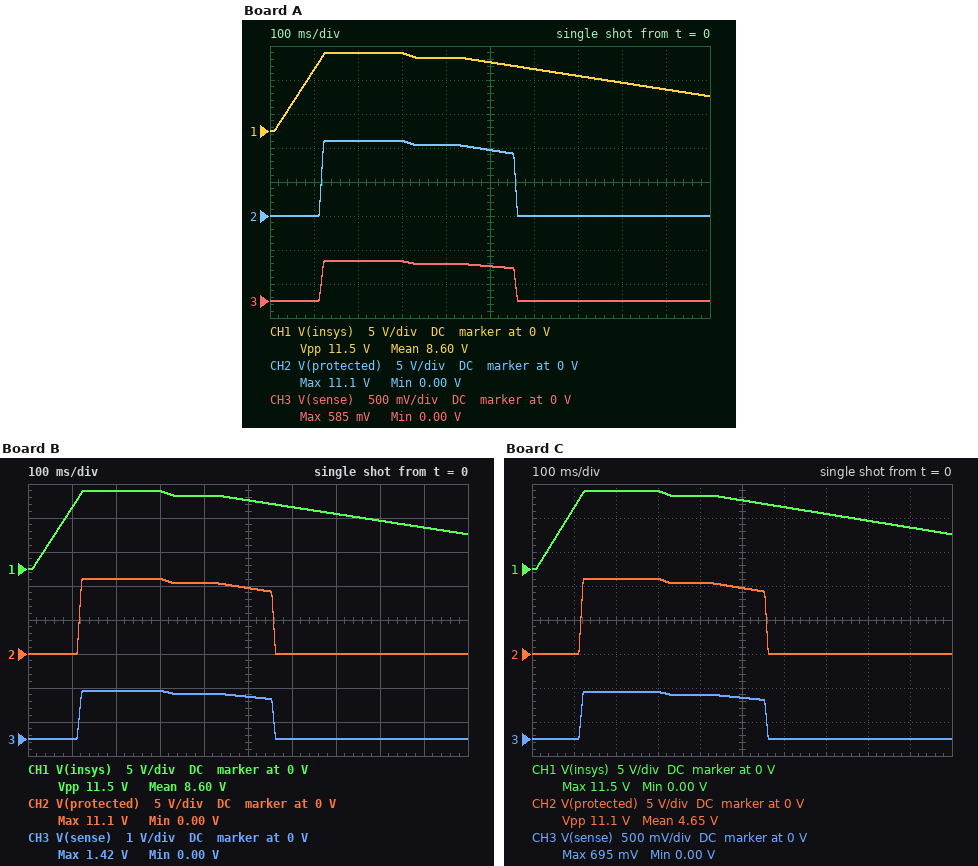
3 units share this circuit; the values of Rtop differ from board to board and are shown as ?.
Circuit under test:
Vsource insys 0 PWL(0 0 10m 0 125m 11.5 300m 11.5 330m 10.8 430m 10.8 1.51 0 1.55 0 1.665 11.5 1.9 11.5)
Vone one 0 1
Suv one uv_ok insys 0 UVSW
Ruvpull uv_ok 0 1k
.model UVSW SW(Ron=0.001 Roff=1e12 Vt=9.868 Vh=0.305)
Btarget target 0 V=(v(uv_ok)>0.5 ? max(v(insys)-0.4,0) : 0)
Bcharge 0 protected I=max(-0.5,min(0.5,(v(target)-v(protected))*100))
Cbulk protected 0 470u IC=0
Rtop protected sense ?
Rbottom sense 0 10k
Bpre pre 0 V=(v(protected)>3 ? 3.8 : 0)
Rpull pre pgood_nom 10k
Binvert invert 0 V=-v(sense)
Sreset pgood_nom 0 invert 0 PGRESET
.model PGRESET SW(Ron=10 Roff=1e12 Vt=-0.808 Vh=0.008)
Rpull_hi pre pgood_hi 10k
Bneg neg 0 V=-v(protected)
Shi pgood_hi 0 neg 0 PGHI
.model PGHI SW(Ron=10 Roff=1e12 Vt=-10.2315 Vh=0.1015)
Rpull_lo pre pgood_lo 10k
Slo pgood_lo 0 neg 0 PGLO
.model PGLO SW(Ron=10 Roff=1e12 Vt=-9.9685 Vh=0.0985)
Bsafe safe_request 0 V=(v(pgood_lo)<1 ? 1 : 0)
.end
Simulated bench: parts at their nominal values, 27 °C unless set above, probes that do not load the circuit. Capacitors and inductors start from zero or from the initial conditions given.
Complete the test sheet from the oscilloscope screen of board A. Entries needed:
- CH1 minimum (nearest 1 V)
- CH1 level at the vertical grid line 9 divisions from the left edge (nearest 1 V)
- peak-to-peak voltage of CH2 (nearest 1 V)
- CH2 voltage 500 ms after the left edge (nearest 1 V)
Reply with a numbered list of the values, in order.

1. 0 V
2. 6 V
3. 11 V
4. 10 V
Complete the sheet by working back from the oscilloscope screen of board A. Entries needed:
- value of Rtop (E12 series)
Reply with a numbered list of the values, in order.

1. 180 kΩ
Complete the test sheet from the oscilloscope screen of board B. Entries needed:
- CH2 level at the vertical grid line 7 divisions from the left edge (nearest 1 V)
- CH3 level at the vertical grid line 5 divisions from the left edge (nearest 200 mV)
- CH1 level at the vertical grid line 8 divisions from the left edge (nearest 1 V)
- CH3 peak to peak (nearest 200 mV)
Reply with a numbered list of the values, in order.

1. 0 V
2. 1.2 V
3. 7 V
4. 1.4 V
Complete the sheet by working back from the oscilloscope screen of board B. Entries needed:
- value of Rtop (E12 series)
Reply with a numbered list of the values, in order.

1. 68 kΩ
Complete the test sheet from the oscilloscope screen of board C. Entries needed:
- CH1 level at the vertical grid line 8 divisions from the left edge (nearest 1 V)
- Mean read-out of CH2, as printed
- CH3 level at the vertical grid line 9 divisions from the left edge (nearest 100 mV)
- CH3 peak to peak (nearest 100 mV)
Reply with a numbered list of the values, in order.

1. 7 V
2. 4.65 V
3. 0 V
4. 700 mV
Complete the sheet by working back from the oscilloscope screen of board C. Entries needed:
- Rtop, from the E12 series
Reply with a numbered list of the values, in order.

1. 150 kΩ
